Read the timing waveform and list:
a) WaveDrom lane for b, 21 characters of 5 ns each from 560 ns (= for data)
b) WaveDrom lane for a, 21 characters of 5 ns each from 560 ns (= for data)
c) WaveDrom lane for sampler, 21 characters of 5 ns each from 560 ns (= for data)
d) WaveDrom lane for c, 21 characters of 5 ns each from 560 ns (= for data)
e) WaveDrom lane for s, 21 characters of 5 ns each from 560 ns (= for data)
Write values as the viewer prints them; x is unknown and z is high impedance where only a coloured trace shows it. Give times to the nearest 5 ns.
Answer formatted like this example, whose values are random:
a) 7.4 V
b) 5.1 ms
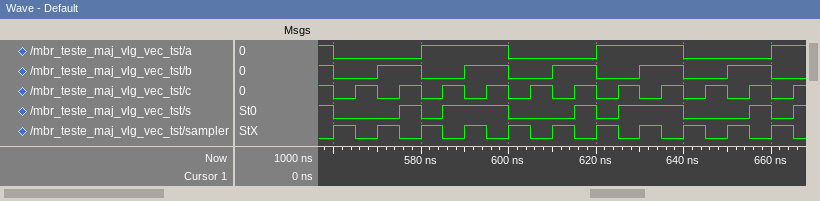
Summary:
a) {name: 'b', wave: '0.1.0.1.0.1.0.1.0.1.0'}
b) {name: 'a', wave: '0...1...0...1...0...1'}
c) {name: 'sampler', wave: '101010101010101010101'}
d) {name: 'c', wave: '010101010101010101010'}
e) {name: 's', wave: '0..101..0..101..0..10'}
